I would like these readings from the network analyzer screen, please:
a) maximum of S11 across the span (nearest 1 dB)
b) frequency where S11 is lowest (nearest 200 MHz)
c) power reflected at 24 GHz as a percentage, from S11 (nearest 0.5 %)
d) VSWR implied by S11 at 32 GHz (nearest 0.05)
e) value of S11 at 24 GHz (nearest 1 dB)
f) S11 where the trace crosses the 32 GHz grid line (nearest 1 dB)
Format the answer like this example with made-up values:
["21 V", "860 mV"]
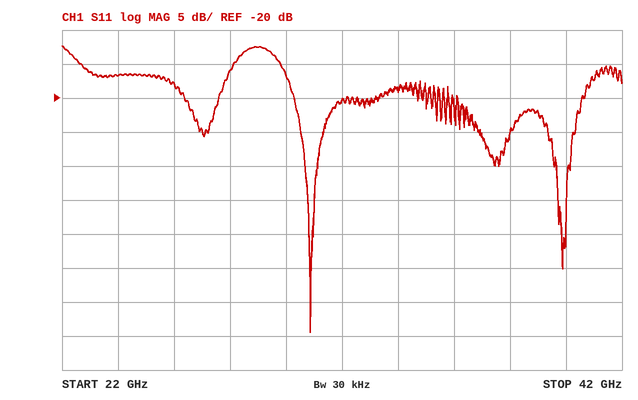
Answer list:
["-12 dB", "30.8 GHz", "2.0 %", "1.20", "-17 dB", "-20 dB"]
